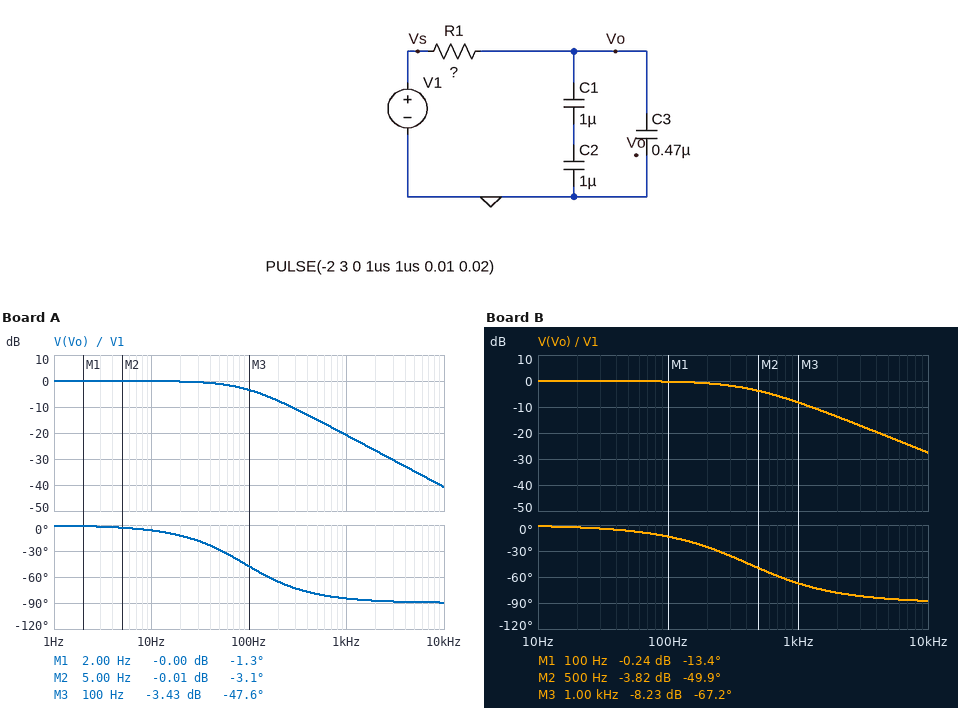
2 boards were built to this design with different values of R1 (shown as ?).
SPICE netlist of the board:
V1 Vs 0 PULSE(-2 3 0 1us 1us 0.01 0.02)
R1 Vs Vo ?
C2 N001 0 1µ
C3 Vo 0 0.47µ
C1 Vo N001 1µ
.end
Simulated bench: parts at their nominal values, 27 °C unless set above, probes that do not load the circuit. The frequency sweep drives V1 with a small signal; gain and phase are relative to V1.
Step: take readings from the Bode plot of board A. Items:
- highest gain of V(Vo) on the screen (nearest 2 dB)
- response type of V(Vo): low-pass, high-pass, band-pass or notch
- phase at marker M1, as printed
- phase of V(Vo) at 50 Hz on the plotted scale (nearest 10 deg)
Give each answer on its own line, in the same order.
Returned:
0 dB
low-pass
-1.3 deg
-30 deg
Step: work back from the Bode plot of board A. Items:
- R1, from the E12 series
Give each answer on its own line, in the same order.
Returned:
1.8 kΩ
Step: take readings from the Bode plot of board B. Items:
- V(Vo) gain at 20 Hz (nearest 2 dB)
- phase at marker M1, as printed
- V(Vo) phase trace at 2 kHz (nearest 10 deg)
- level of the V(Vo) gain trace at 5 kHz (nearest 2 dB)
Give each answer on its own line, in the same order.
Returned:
0 dB
-13.4 deg
-80 deg
-22 dB
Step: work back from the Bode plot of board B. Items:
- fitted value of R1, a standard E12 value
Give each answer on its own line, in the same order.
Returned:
390 Ω
